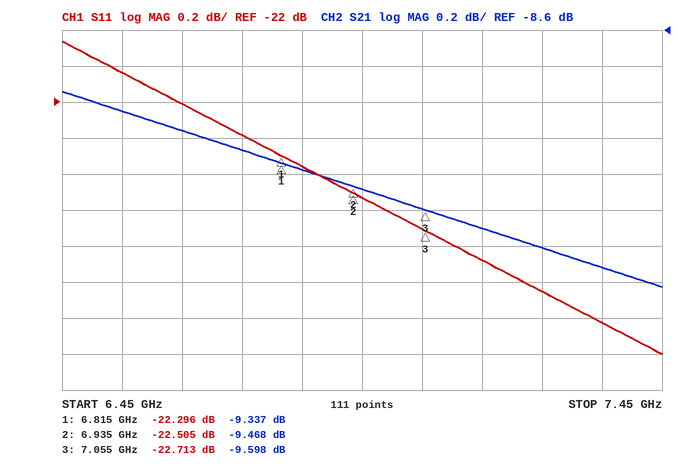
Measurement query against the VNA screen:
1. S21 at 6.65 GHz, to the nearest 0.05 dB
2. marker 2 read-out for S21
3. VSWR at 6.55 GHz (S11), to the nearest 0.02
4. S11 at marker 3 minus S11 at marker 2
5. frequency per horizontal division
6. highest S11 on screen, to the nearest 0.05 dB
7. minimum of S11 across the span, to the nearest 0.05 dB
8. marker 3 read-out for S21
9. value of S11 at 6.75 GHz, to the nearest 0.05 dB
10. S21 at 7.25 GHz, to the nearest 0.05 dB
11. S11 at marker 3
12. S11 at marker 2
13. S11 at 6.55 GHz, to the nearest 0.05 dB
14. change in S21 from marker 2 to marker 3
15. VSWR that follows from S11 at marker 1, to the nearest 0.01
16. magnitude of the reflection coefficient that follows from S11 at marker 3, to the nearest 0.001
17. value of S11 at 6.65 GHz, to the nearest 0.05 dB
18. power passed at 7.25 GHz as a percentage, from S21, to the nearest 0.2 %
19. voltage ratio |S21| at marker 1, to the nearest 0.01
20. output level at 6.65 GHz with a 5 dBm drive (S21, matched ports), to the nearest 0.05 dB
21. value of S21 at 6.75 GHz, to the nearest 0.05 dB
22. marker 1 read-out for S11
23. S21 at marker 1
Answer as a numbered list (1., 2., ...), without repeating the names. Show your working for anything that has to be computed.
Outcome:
1. -9.15 dB
2. -9.468 dB
3. |Γ| = 10^(-21.85/20) = 0.0808; VSWR = (1 + 0.0808)/(1 − 0.0808) ≈ 1.18
4. -22.713 − (-22.505) = -0.208 dB
5. 100 MHz
6. -21.65 dB
7. -23.40 dB
8. -9.598 dB
9. -22.20 dB
10. -9.80 dB
11. -22.713 dB
12. -22.505 dB
13. -21.85 dB
14. -9.598 − (-9.468) = -0.130 dB
15. (1 + 0.0768)/(1 − 0.0768) ≈ 1.17
16. 10^(-22.713/20) ≈ 0.073
17. -22.00 dB
18. 10^(-9.8/10) ≈ 10.5 %, so 10.4 % to the nearest 0.2 %
19. 10^(-9.337/20) ≈ 0.34
20. 5 dBm + (-9.15 dB) = -4.15 dBm
21. -9.25 dB
22. -22.296 dB
23. -9.337 dB
